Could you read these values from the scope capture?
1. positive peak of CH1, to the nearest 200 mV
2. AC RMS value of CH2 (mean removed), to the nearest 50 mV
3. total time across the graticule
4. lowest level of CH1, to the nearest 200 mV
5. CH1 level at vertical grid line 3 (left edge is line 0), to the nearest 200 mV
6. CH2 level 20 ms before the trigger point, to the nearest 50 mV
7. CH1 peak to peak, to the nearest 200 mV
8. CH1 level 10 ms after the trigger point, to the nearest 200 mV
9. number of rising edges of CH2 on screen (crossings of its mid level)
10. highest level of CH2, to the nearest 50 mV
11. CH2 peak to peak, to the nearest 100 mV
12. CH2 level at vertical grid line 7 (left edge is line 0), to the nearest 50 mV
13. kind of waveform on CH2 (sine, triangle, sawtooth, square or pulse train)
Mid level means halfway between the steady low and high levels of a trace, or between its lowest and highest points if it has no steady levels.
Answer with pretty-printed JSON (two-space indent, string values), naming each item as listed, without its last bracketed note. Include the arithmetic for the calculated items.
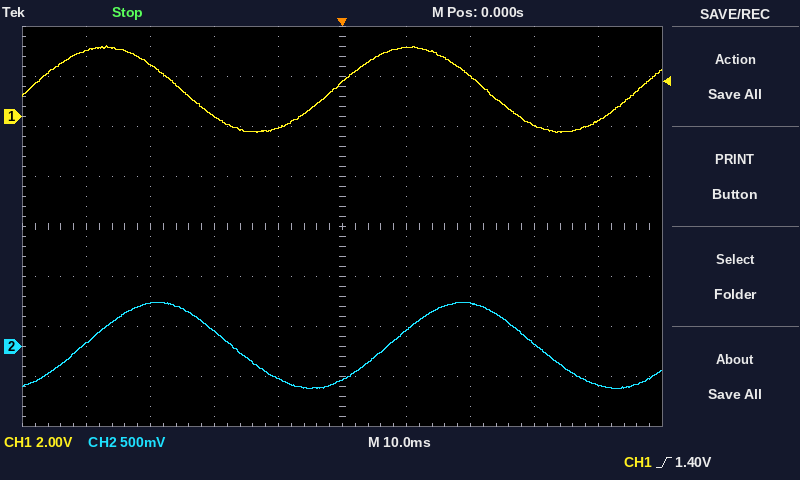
{
  "positive peak of CH1, to the nearest 200 mV": "2.8 V",
  "AC RMS value of CH2 (mean removed), to the nearest 50 mV": "900 mV / (2√2) ≈ 318 mV, so 300 mV to the nearest 50 mV",
  "total time across the graticule": "100 ms",
  "lowest level of CH1, to the nearest 200 mV": "-600 mV",
  "CH1 level at vertical grid line 3 (left edge is line 0), to the nearest 200 mV": "0.0 V",
  "CH2 level 20 ms before the trigger point, to the nearest 50 mV": "150 mV",
  "CH1 peak to peak, to the nearest 200 mV": "2.8 V − (-600 mV) = 3.4 V",
  "CH1 level 10 ms after the trigger point, to the nearest 200 mV": "2.8 V",
  "number of rising edges of CH2 on screen": "2",
  "highest level of CH2, to the nearest 50 mV": "450 mV",
  "CH2 peak to peak, to the nearest 100 mV": "900 mV",
  "CH2 level at vertical grid line 7 (left edge is line 0), to the nearest 50 mV": "450 mV",
  "kind of waveform on CH2": "sine"
}
